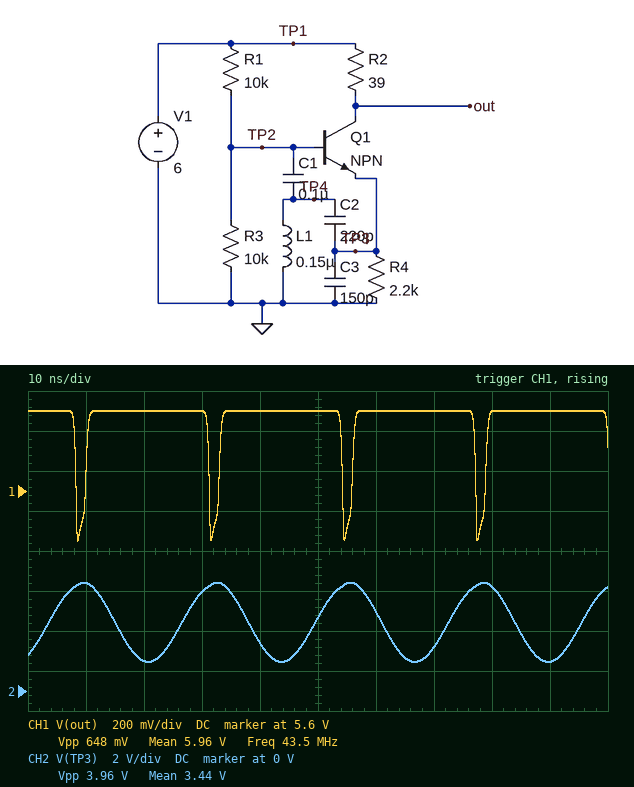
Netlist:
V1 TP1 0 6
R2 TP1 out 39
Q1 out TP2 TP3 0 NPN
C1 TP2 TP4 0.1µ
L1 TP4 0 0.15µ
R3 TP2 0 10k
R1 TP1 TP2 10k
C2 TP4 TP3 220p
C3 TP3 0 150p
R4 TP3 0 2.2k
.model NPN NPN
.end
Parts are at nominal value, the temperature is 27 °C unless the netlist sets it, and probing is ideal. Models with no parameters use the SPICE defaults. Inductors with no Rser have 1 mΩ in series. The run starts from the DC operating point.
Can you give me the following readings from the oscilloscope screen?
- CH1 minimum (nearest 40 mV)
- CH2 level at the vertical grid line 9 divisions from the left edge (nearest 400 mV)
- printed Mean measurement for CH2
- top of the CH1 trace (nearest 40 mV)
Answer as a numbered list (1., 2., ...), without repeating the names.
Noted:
1. 5.36 V
2. 1.6 V
3. 3.44 V
4. 6.00 V
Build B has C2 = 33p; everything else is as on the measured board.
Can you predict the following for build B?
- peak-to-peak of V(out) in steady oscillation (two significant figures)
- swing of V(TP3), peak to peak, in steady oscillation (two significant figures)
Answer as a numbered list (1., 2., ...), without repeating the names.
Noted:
1. 1.4 V
2. 970 mV
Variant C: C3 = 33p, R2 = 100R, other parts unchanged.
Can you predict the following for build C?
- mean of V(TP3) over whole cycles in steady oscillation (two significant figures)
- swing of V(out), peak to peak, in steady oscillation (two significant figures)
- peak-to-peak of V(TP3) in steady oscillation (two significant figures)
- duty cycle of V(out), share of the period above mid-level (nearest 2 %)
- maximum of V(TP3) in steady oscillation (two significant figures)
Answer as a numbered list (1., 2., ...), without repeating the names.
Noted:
1. 2.5 V
2. 860 mV
3. 5.4 V
4. 88 %
5. 5.2 V
